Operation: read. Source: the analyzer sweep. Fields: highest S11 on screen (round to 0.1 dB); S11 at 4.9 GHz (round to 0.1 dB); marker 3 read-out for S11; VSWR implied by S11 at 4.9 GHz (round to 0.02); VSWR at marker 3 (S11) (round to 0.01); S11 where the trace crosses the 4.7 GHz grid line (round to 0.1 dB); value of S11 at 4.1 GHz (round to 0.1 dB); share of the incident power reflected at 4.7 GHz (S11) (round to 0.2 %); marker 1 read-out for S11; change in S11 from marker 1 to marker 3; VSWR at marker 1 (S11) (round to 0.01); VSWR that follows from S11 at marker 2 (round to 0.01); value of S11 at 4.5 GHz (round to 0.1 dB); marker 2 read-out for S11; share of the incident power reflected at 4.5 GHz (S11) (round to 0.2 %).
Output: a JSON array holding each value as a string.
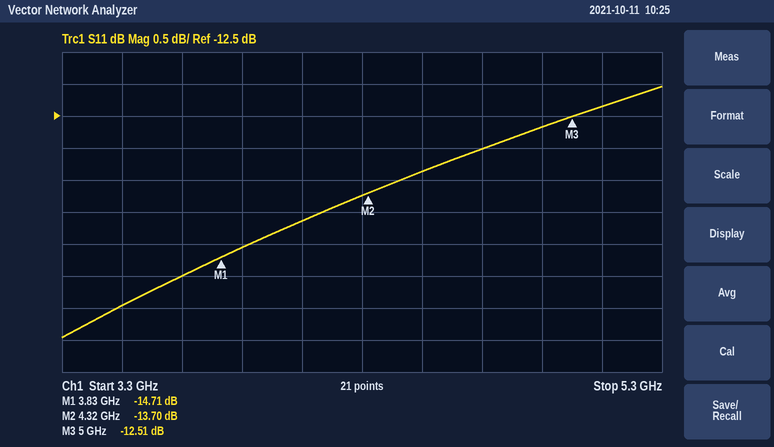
["-12.0 dB", "-12.7 dB", "-12.51 dB", "1.60", "1.62", "-13.0 dB", "-14.1 dB", "5.0 %", "-14.71 dB", "2.20 dB", "1.45", "1.52", "-13.4 dB", "-13.70 dB", "4.6 %"]
